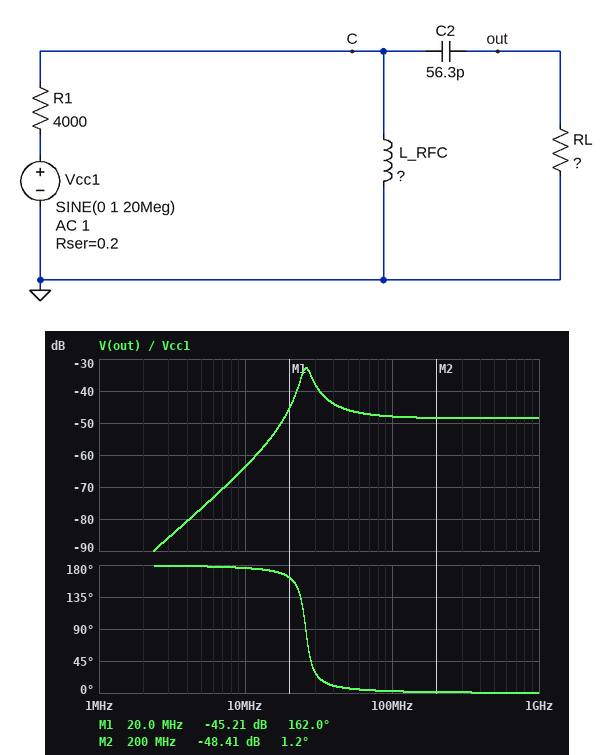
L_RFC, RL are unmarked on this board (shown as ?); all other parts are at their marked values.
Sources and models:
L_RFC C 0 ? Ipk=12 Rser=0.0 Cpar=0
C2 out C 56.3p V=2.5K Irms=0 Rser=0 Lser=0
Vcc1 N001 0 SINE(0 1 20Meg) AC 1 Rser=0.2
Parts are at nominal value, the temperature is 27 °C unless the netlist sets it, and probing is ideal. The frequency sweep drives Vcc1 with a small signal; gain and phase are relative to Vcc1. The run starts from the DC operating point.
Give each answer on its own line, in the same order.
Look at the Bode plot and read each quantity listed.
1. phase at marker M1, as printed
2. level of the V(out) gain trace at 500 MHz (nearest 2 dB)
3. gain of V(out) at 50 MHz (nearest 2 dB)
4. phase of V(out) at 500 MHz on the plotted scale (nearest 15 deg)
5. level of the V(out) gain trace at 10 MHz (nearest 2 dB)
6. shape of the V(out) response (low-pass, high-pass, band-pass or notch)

162.0 deg
-48 dB
-46 dB
0 deg
-64 dB
high-pass
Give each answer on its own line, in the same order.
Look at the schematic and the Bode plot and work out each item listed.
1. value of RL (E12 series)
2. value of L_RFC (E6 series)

15 Ω
680 nH
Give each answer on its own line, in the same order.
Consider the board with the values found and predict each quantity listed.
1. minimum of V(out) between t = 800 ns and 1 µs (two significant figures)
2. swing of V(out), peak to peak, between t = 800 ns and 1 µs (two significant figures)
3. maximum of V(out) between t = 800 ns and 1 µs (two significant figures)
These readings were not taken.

-5.5 mV
11 mV
5.5 mV
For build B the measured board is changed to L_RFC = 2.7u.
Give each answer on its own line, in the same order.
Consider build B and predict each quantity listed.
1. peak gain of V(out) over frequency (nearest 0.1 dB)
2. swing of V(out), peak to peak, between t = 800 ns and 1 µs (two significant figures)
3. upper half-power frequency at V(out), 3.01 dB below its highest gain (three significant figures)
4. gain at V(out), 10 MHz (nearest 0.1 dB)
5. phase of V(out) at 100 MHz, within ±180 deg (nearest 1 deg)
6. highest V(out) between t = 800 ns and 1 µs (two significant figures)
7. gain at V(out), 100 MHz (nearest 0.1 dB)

-30.3 dB
13 mV
13.8 MHz
-45.2 dB
1 deg
6.4 mV
-48.4 dB
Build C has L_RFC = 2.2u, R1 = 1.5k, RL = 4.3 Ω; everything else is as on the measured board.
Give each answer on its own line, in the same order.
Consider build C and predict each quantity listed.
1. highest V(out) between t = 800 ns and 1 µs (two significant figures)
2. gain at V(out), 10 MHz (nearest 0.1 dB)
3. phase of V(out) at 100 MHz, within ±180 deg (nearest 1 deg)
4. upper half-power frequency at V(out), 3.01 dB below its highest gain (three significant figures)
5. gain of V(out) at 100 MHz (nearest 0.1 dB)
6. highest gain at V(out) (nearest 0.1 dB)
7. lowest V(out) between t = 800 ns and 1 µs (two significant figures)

5.7 mV
-51.4 dB
1 deg
15.6 MHz
-50.7 dB
-34.6 dB
-5.7 mV
